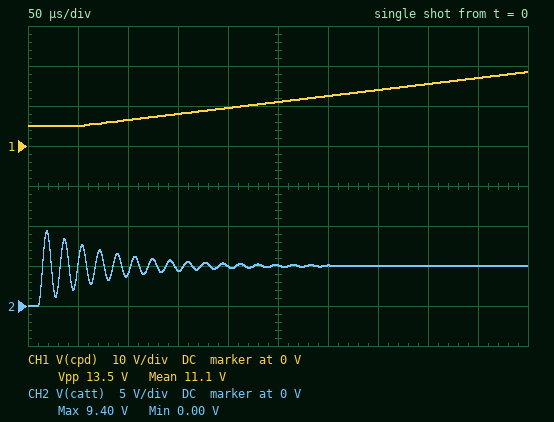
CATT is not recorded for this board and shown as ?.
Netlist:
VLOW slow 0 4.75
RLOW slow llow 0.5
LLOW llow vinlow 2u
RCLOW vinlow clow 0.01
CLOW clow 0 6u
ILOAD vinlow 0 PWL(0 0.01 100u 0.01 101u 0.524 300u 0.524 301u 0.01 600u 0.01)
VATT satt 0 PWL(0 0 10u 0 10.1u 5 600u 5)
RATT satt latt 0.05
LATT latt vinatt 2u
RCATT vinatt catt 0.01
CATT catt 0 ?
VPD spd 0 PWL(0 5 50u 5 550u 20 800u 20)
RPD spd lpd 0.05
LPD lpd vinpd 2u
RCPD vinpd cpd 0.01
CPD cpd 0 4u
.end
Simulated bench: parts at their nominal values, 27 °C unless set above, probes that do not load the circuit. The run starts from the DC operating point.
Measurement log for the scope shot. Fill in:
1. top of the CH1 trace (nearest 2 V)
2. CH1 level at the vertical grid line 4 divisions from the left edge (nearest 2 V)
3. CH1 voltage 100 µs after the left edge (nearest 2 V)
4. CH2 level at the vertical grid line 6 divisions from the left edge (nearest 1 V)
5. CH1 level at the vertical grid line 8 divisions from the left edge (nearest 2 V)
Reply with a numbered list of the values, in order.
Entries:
1. 18 V
2. 10 V
3. 6 V
4. 5 V
5. 16 V
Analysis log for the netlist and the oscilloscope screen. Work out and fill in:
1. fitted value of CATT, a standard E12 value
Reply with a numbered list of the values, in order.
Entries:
1. 3.9 µF
